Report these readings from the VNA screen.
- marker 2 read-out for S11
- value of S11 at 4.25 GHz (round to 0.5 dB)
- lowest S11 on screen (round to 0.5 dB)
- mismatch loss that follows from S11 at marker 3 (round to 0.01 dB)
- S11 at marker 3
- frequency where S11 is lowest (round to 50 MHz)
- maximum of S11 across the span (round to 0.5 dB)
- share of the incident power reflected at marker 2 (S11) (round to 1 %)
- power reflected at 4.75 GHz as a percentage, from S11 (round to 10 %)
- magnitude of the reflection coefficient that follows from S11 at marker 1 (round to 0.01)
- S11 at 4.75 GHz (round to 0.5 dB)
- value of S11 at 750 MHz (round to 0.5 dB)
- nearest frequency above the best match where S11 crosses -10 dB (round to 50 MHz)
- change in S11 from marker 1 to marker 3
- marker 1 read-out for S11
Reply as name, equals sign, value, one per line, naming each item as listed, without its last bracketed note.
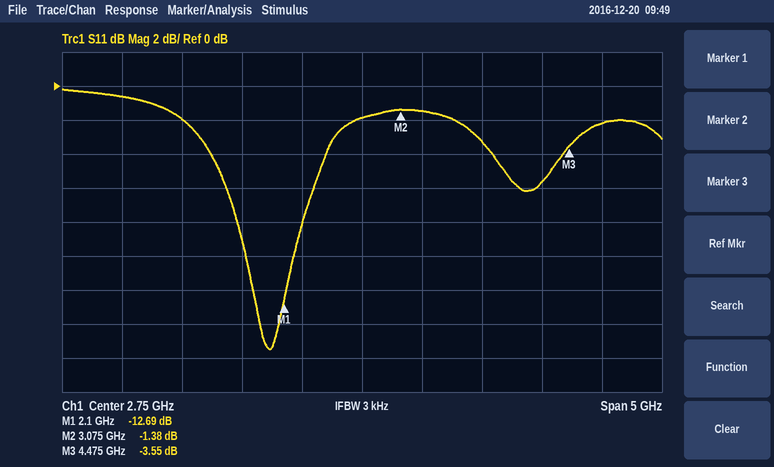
marker 2 read-out for S11 = -1.38 dB
value of S11 at 4.25 GHz = -5.5 dB
lowest S11 on screen = -15.5 dB
mismatch loss that follows from S11 at marker 3 = 2.53 dB
S11 at marker 3 = -3.55 dB
frequency where S11 is lowest = 2.00 GHz
maximum of S11 across the span = 0.0 dB
share of the incident power reflected at marker 2 (S11) = 73 %
power reflected at 4.75 GHz as a percentage, from S11 = 60 %
magnitude of the reflection coefficient that follows from S11 at marker 1 = 0.23
S11 at 4.75 GHz = -2.0 dB
value of S11 at 750 MHz = -0.5 dB
nearest frequency above the best match where S11 crosses -10 dB = 2.20 GHz
change in S11 from marker 1 to marker 3 = 9.14 dB
marker 1 read-out for S11 = -12.69 dB
